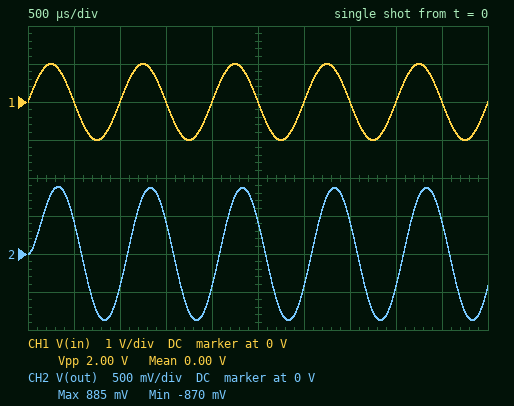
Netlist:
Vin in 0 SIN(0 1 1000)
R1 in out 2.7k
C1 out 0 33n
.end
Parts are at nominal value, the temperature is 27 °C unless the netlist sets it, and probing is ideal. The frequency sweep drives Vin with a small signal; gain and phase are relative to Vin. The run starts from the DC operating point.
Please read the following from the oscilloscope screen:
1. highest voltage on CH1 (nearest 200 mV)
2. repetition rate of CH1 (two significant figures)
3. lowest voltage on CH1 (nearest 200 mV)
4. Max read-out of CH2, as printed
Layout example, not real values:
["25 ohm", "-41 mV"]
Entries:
["1.0 V", "1.0 kHz", "-1.0 V", "885 mV"]
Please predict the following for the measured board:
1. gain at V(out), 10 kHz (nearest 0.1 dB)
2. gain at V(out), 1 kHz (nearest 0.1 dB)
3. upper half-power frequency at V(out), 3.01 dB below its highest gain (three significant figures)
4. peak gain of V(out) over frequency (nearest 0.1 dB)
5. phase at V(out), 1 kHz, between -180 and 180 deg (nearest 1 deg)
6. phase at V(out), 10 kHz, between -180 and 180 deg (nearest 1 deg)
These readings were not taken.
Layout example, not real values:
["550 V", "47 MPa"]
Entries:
["-15.1 dB", "-1.2 dB", "1.79 kHz", "0 dB", "-29 deg", "-80 deg"]
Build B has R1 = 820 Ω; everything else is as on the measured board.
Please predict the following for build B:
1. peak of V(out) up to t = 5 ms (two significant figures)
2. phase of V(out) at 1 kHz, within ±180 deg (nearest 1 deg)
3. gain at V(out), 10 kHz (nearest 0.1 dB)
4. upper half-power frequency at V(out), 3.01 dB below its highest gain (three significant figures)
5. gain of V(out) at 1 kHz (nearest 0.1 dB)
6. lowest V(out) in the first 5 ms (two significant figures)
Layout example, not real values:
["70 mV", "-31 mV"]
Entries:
["990 mV", "-10 deg", "-5.9 dB", "5.88 kHz", "-0.1 dB", "-990 mV"]
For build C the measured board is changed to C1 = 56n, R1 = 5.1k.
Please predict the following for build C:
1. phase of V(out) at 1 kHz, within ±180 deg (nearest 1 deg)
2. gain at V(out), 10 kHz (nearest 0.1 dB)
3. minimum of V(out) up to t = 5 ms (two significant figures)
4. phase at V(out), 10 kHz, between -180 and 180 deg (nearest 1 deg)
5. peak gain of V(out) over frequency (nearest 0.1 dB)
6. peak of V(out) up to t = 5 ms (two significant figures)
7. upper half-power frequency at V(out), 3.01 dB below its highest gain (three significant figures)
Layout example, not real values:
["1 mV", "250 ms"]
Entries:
["-61 deg", "-25.1 dB", "-490 mV", "-87 deg", "0 dB", "590 mV", "557 Hz"]
